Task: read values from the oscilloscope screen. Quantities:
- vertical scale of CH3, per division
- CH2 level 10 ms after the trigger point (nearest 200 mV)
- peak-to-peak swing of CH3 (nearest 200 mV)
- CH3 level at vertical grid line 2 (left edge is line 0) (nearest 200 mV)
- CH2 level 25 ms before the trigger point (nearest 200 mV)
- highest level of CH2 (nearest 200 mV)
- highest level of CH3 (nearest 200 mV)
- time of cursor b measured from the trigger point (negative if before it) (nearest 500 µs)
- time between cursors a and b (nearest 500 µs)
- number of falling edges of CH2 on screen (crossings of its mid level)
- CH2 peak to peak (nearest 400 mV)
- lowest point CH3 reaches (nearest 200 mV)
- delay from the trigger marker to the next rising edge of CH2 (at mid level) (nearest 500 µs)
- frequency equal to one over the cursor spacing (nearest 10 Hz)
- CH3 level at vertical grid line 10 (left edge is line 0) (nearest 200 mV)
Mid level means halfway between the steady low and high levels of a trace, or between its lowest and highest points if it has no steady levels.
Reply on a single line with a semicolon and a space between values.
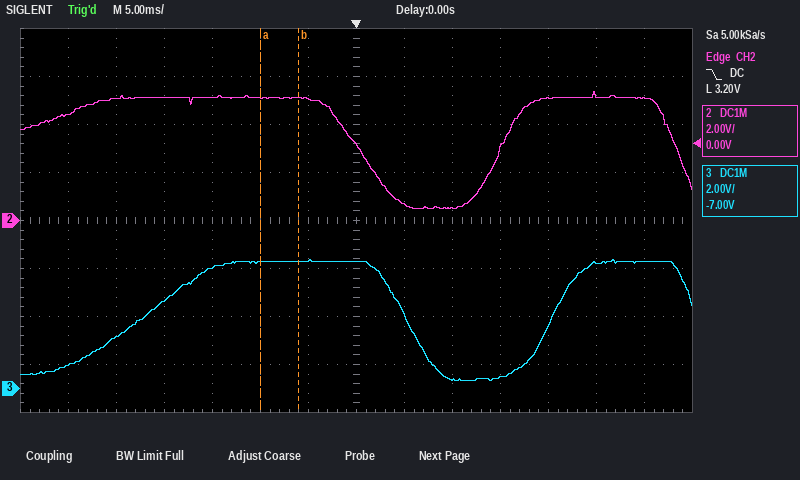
2 V; 600 mV; 5.0 V; 2.2 V; 5.0 V; 5.4 V; 5.4 V; -6.0 ms; 4.0 ms; 2; 4.8 V; 400 mV; 15.0 ms; 250 Hz; 400 mV
